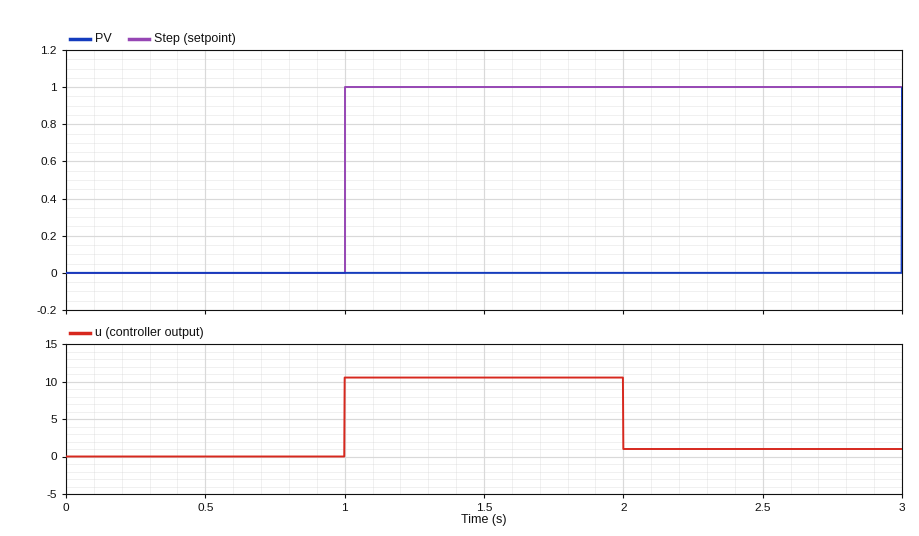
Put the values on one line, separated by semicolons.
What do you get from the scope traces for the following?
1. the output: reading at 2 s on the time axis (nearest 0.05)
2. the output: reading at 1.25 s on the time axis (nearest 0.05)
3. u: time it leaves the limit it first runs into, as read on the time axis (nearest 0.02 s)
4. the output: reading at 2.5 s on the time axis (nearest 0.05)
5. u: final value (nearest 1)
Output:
0.00; 0.00; 2.00 s; 0.00; 1
